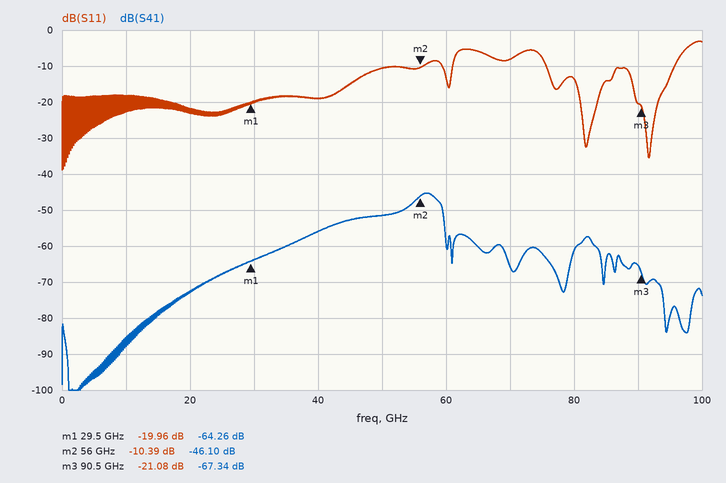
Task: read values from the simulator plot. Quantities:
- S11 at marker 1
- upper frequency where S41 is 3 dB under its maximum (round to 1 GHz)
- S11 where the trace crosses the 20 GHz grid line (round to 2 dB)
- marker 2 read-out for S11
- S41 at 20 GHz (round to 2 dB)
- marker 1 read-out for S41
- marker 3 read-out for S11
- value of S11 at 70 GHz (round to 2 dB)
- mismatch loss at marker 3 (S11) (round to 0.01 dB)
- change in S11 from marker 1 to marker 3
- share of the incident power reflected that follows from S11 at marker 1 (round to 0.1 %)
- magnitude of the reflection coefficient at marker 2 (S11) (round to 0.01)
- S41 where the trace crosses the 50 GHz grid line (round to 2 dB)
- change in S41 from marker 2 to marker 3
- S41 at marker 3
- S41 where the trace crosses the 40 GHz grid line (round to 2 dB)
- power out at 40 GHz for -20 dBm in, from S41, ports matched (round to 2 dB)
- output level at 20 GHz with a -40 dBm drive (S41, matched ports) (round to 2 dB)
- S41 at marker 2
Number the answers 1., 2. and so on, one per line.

1. -19.96 dB
2. 59 GHz
3. -22 dB
4. -10.39 dB
5. -72 dB
6. -64.26 dB
7. -21.08 dB
8. -8 dB
9. 0.03 dB
10. -1.12 dB
11. 1.0 %
12. 0.30
13. -52 dB
14. -21.24 dB
15. -67.34 dB
16. -56 dB
17. -76 dBm
18. -112 dBm
19. -46.10 dB
